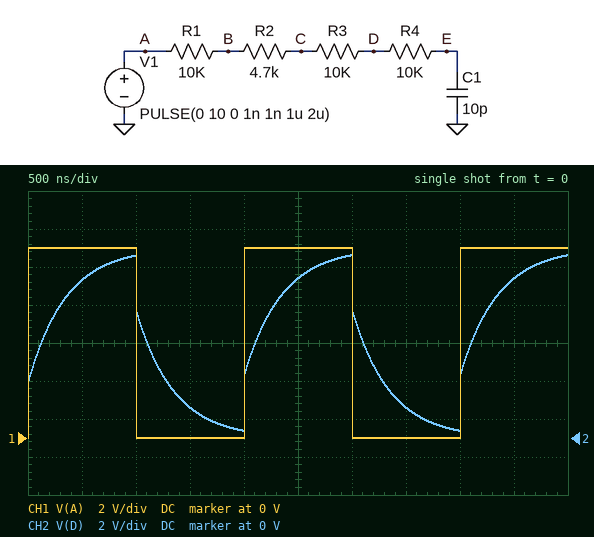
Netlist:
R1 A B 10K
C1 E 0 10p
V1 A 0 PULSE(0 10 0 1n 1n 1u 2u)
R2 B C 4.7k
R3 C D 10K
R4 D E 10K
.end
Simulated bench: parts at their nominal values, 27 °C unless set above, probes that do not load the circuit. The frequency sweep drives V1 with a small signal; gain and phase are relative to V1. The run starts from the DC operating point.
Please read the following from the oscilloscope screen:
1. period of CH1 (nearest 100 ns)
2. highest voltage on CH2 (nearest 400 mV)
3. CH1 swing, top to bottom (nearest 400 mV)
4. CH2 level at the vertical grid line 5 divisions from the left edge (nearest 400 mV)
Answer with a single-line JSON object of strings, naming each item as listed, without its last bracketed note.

{"period of CH1": "2.0 µs", "highest voltage on CH2": "9.6 V", "CH1 swing, top to bottom": "10.0 V", "CH2 level at the vertical grid line 5 divisions from the left edge": "8.4 V"}
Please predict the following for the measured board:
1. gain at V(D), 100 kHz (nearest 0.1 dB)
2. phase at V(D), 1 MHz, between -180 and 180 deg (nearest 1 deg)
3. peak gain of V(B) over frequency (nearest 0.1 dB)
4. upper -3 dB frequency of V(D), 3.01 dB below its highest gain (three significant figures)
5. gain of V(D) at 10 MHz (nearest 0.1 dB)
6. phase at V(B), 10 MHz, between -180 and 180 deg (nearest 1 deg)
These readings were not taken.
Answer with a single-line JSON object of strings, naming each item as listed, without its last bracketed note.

{"gain at V(D), 100 kHz": "-0.2 dB", "phase at V(D), 1 MHz, between -180 and 180 deg": "-33 deg", "peak gain of V(B) over frequency": "0 dB", "upper -3 dB frequency of V(D), 3.01 dB below its highest gain": "502 kHz", "gain of V(D) at 10 MHz": "-10.7 dB", "phase at V(B), 10 MHz, between -180 and 180 deg": "-1 deg"}
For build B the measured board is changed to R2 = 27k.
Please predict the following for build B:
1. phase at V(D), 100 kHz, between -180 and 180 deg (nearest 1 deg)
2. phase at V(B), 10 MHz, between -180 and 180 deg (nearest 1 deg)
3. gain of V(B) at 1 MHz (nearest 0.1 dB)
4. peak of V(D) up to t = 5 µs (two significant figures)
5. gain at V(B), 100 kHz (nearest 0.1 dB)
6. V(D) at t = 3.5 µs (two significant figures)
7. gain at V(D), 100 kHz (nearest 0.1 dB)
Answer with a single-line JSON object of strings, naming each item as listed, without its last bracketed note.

{"phase at V(D), 100 kHz, between -180 and 180 deg": "-16 deg", "phase at V(B), 10 MHz, between -180 and 180 deg": "0 deg", "gain of V(B) at 1 MHz": "-1.5 dB", "peak of V(D) up to t = 5 µs": "8.8 V", "gain at V(B), 100 kHz": "-0.2 dB", "V(D) at t = 3.5 µs": "2.9 V", "gain at V(D), 100 kHz": "-0.5 dB"}
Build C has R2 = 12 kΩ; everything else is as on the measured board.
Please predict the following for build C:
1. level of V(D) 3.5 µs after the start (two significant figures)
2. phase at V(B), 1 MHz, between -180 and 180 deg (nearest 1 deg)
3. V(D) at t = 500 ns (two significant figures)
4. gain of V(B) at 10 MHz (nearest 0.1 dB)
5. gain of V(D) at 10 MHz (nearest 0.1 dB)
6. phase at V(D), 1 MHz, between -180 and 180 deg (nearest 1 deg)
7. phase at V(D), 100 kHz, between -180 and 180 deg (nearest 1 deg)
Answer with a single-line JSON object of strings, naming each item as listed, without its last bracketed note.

{"level of V(D) 3.5 µs after the start": "2.1 V", "phase at V(B), 1 MHz, between -180 and 180 deg": "-6 deg", "V(D) at t = 500 ns": "7.7 V", "gain of V(B) at 10 MHz": "-2.4 dB", "gain of V(D) at 10 MHz": "-12.4 dB", "phase at V(D), 1 MHz, between -180 and 180 deg": "-37 deg", "phase at V(D), 100 kHz, between -180 and 180 deg": "-11 deg"}
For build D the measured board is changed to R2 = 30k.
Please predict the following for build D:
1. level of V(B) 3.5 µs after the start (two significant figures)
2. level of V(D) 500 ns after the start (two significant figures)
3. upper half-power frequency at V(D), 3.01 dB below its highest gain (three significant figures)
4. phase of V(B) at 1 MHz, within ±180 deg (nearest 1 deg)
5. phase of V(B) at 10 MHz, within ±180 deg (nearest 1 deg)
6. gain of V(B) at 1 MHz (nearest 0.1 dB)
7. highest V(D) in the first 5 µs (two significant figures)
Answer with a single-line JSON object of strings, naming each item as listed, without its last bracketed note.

{"level of V(B) 3.5 µs after the start": "610 mV", "level of V(D) 500 ns after the start": "6.4 V", "upper half-power frequency at V(D), 3.01 dB below its highest gain": "273 kHz", "phase of V(B) at 1 MHz, within ±180 deg": "-3 deg", "phase of V(B) at 10 MHz, within ±180 deg": "0 deg", "gain of V(B) at 1 MHz": "-1.5 dB", "highest V(D) in the first 5 µs": "8.7 V"}
